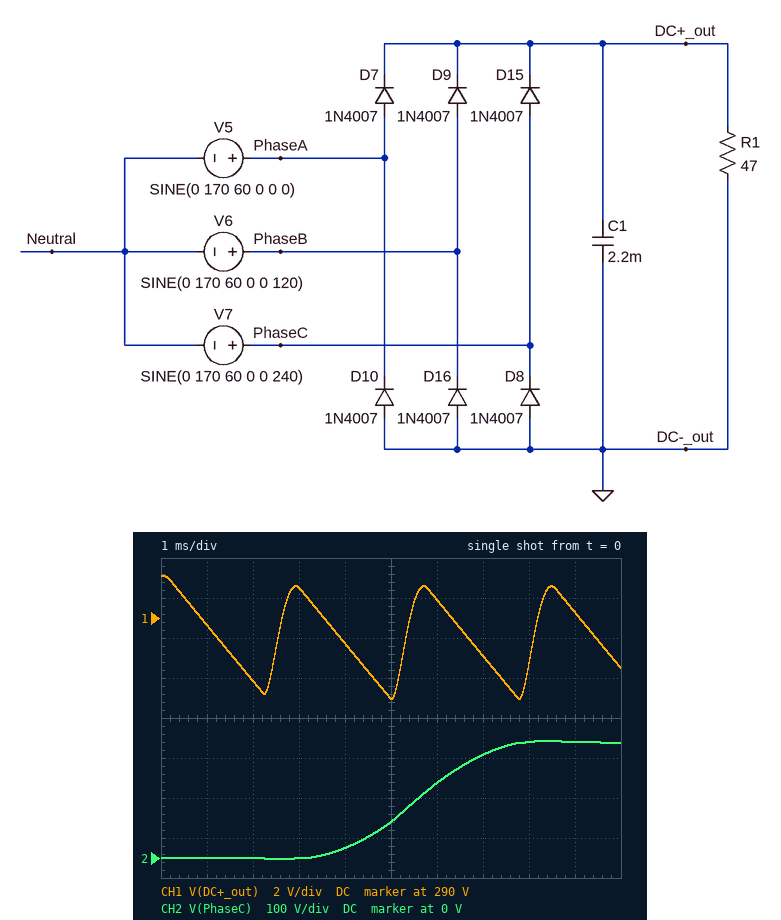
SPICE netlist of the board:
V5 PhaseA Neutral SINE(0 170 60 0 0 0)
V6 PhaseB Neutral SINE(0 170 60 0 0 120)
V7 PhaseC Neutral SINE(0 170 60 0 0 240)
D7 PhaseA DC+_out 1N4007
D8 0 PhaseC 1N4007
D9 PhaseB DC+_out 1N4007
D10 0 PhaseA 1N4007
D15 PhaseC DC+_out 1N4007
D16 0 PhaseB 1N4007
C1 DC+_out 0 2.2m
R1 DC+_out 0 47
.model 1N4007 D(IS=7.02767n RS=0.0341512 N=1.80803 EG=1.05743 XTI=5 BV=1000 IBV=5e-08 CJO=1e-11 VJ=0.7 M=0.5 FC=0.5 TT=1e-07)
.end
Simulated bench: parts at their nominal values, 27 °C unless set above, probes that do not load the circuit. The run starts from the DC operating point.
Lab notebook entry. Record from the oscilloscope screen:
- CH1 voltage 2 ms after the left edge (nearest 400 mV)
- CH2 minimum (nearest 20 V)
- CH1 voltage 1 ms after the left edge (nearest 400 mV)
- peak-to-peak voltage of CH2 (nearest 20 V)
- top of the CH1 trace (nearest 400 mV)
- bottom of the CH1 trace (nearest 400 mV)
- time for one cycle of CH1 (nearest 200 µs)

286.8 V
0 V
289.6 V
300 V
292.0 V
286.0 V
2.8 ms
